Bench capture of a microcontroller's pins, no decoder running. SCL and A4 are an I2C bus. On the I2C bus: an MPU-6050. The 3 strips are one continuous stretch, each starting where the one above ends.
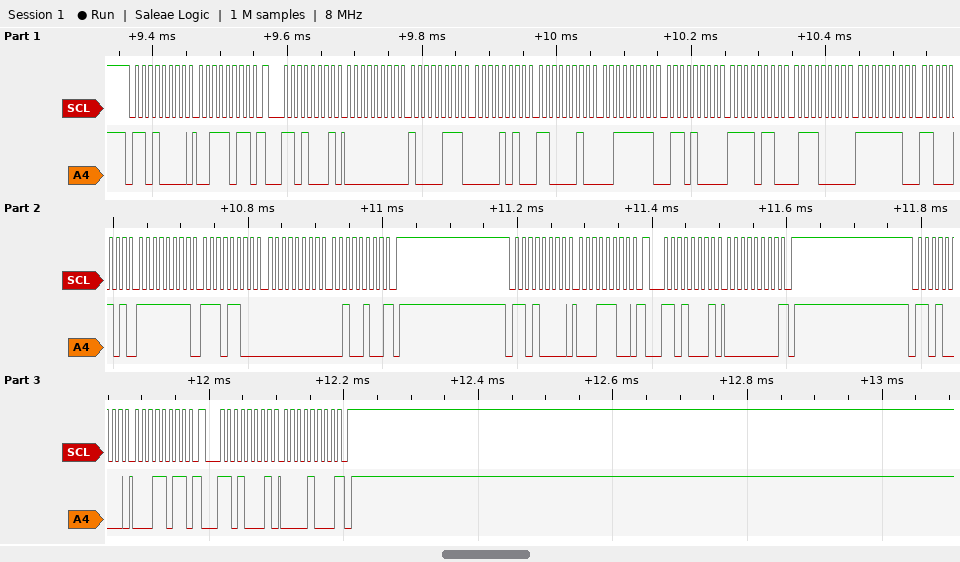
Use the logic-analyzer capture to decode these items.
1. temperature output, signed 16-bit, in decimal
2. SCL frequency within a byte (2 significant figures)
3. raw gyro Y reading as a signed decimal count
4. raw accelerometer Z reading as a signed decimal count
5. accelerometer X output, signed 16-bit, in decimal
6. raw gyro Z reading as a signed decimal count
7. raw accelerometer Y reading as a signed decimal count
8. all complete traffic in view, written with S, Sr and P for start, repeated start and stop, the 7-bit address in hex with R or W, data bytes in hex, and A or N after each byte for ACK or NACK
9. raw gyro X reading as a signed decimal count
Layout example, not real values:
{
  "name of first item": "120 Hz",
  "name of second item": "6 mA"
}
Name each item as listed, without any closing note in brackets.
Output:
{
  "temperature output, signed 16-bit, in decimal": "-2448",
  "SCL frequency within a byte": "100 kHz",
  "raw gyro Y reading as a signed decimal count": "-20",
  "raw accelerometer Z reading as a signed decimal count": "16232",
  "accelerometer X output, signed 16-bit, in decimal": "135",
  "raw gyro Z reading as a signed decimal count": "36",
  "raw accelerometer Y reading as a signed decimal count": "2754",
  "all complete traffic in view, written with S, Sr and P for start, repeated start and stop, the 7-bit address in hex with R or W, data bytes in hex, and A or N after each byte for ACK or NACK": "S 68W A 3B A Sr 68R A 00 A 87 A 0A A C2 A 3F A 68 A F6 A 70 A FE A C5 A FF A EC A 00 A 24 N P S 68W A 1C A Sr 68R A 00 N P S 68W A 1B A Sr 68R A 08 N P",
  "raw gyro X reading as a signed decimal count": "-315"
}
